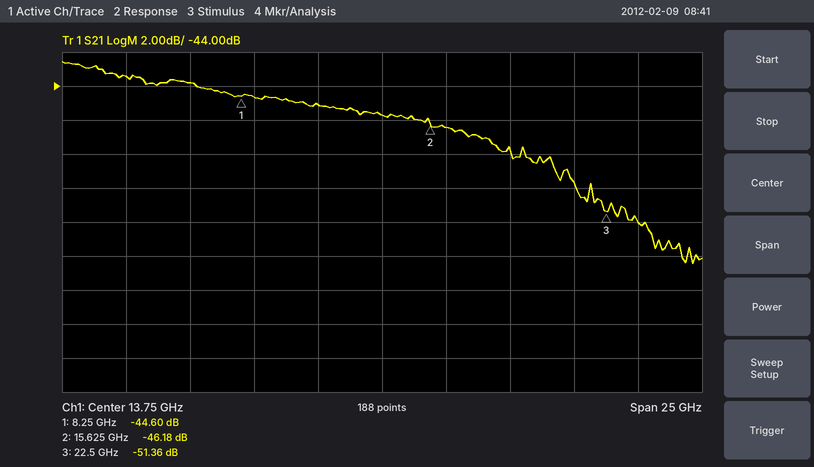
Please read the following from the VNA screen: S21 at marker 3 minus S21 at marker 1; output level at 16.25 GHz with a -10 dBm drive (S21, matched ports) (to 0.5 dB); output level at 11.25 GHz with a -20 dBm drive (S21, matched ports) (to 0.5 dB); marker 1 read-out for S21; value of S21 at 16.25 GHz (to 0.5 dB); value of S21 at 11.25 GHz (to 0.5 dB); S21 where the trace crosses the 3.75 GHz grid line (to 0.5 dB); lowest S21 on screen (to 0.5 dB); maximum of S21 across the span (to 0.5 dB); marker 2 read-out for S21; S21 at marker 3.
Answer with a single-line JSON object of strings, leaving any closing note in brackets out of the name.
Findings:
{"S21 at marker 3 minus S21 at marker 1": "-6.76 dB", "output level at 16.25 GHz with a -10 dBm drive (S21, matched ports)": "-56.5 dBm", "output level at 11.25 GHz with a -20 dBm drive (S21, matched ports)": "-65.0 dBm", "marker 1 read-out for S21": "-44.60 dB", "value of S21 at 16.25 GHz": "-46.5 dB", "value of S21 at 11.25 GHz": "-45.0 dB", "S21 where the trace crosses the 3.75 GHz grid line": "-43.5 dB", "lowest S21 on screen": "-54.5 dB", "maximum of S21 across the span": "-42.5 dB", "marker 2 read-out for S21": "-46.18 dB", "S21 at marker 3": "-51.36 dB"}
